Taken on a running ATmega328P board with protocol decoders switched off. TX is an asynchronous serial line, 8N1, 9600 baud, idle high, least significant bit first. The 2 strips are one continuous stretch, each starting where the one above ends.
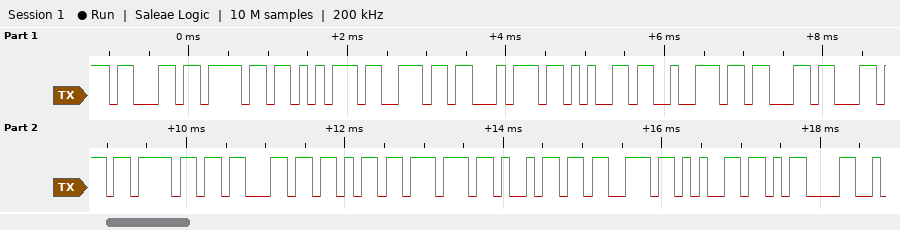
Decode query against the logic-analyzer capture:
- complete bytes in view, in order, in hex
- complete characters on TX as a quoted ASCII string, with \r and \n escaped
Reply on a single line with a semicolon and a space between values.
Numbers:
0x63 0x6F 0x75 0x6E 0x74 0x65 0x72 0x63 0x6C 0x6F 0x63 0x6B 0x77 0x69 0x73 0x65 0x0D; "counterclockwise\r"
